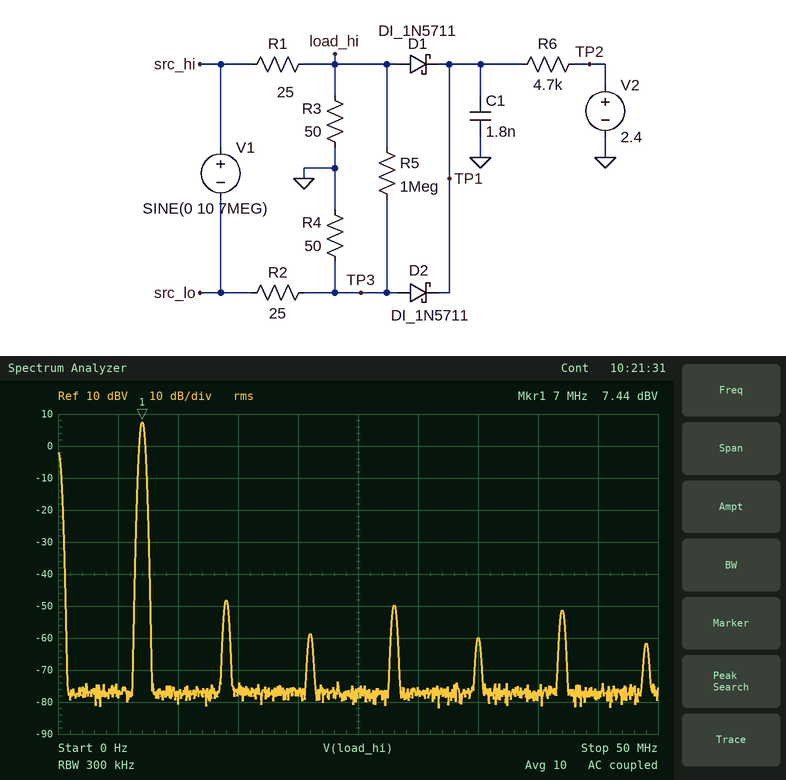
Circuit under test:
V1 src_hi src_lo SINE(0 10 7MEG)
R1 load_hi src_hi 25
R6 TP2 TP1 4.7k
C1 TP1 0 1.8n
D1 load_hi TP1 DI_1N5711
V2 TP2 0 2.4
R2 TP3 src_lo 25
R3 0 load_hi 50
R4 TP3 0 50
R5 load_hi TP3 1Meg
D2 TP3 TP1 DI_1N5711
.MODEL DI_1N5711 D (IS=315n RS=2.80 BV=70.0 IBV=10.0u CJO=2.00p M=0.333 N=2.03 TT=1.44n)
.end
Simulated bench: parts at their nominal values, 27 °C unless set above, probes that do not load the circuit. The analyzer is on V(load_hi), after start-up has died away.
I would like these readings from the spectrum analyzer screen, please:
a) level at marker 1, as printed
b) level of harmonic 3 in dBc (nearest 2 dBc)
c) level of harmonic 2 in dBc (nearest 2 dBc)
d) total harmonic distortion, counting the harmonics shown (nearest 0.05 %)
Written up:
7.44 dBV
-66 dBc
-56 dBc
0.25 %
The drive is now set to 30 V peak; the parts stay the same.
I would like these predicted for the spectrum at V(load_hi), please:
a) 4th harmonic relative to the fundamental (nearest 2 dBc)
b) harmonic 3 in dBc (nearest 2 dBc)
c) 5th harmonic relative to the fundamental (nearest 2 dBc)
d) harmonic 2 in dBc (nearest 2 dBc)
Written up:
-44 dBc
-54 dBc
-54 dBc
-44 dBc
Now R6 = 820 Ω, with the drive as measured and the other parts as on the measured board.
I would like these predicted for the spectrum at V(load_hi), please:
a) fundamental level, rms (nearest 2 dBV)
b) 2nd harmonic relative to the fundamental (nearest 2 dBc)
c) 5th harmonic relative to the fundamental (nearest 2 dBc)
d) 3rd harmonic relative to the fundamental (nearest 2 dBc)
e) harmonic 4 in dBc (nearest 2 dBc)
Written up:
8 dBV
-44 dBc
-56 dBc
-54 dBc
-46 dBc
